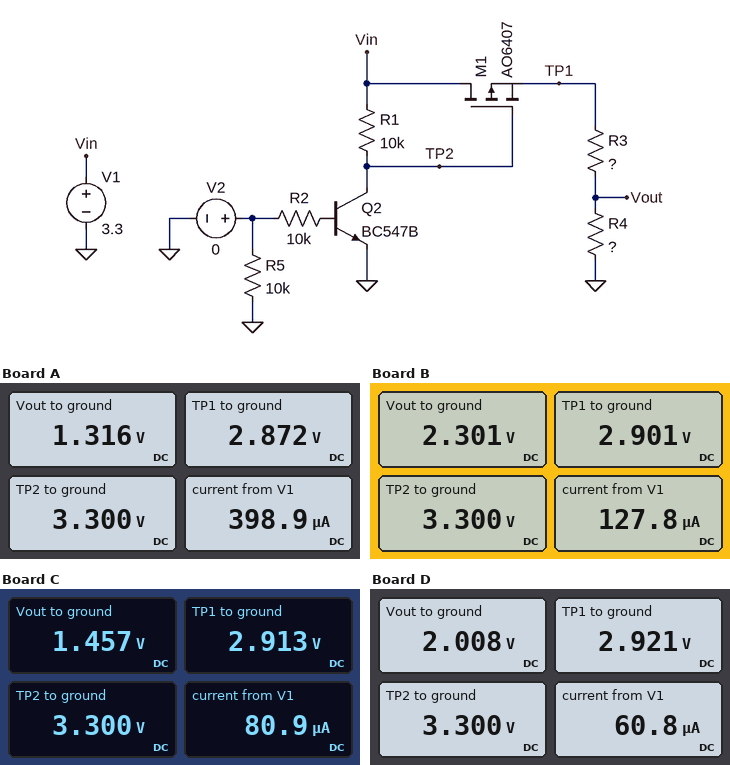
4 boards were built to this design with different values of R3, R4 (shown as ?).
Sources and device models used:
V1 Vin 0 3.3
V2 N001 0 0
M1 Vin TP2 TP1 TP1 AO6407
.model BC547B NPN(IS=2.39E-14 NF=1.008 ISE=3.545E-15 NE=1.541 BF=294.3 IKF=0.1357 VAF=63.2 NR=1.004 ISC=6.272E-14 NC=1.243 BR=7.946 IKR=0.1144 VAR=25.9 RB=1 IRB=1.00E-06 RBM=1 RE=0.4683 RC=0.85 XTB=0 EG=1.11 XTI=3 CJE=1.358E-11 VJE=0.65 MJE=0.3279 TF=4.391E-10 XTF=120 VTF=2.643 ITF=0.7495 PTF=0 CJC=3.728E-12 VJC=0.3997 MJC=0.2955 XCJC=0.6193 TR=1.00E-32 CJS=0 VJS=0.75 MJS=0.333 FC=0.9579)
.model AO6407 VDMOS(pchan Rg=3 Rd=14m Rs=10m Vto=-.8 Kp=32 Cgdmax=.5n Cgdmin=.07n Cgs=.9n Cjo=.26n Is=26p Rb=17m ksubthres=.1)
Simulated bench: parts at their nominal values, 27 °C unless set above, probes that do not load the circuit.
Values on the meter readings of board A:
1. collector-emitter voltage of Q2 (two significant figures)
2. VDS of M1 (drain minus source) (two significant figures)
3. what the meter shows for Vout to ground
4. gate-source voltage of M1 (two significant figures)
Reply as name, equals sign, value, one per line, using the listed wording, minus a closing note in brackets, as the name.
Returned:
collector-emitter voltage of Q2 = 3.3 V
VDS of M1 (drain minus source) = 430 mV
what the meter shows for Vout to ground = 1.316 V
gate-source voltage of M1 = 430 mV
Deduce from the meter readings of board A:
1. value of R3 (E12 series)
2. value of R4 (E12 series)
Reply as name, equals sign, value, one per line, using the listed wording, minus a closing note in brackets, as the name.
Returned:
value of R3 = 3.9 kΩ
value of R4 = 3.3 kΩ
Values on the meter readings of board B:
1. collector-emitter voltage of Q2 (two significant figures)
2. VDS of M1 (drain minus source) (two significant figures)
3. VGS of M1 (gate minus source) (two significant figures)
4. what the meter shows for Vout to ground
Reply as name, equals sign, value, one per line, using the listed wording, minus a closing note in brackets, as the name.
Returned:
collector-emitter voltage of Q2 = 3.3 V
VDS of M1 (drain minus source) = 400 mV
VGS of M1 (gate minus source) = 400 mV
what the meter shows for Vout to ground = 2.301 V
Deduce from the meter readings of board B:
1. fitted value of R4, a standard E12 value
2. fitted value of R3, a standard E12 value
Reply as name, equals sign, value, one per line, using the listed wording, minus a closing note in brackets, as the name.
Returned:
fitted value of R4, a standard E12 value = 18 kΩ
fitted value of R3, a standard E12 value = 4.7 kΩ
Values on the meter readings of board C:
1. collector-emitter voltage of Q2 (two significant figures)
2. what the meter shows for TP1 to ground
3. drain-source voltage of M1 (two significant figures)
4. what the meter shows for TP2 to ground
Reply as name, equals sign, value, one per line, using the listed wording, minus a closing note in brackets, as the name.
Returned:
collector-emitter voltage of Q2 = 3.3 V
what the meter shows for TP1 to ground = 2.913 V
drain-source voltage of M1 = 390 mV
what the meter shows for TP2 to ground = 3.300 V
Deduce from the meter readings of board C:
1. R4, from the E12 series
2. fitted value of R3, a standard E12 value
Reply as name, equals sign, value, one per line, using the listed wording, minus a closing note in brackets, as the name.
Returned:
R4, from the E12 series = 18 kΩ
fitted value of R3, a standard E12 value = 18 kΩ
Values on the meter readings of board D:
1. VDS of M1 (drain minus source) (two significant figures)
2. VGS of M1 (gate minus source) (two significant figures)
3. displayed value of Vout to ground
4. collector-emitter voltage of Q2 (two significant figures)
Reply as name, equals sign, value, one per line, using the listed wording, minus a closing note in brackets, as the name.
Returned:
VDS of M1 (drain minus source) = 380 mV
VGS of M1 (gate minus source) = 380 mV
displayed value of Vout to ground = 2.008 V
collector-emitter voltage of Q2 = 3.3 V
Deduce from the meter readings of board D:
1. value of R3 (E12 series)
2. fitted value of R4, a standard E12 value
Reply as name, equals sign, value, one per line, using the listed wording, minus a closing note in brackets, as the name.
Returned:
value of R3 = 15 kΩ
fitted value of R4, a standard E12 value = 33 kΩ
